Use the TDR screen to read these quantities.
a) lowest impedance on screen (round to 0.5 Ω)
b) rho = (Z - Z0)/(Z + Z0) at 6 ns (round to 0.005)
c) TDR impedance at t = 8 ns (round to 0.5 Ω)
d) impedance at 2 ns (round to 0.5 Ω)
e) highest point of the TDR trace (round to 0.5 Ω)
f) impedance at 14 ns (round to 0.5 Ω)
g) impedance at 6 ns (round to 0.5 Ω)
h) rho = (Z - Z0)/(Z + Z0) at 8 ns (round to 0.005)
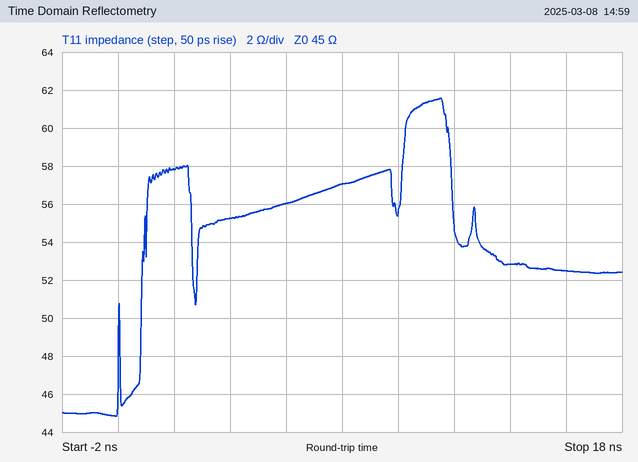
45.0 Ω
+0.110
57.0 Ω
58.0 Ω
61.5 Ω
53.0 Ω
56.0 Ω
+0.120
